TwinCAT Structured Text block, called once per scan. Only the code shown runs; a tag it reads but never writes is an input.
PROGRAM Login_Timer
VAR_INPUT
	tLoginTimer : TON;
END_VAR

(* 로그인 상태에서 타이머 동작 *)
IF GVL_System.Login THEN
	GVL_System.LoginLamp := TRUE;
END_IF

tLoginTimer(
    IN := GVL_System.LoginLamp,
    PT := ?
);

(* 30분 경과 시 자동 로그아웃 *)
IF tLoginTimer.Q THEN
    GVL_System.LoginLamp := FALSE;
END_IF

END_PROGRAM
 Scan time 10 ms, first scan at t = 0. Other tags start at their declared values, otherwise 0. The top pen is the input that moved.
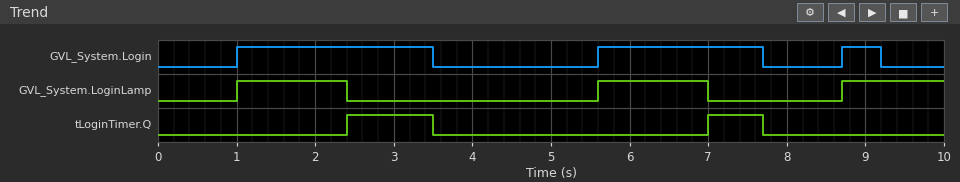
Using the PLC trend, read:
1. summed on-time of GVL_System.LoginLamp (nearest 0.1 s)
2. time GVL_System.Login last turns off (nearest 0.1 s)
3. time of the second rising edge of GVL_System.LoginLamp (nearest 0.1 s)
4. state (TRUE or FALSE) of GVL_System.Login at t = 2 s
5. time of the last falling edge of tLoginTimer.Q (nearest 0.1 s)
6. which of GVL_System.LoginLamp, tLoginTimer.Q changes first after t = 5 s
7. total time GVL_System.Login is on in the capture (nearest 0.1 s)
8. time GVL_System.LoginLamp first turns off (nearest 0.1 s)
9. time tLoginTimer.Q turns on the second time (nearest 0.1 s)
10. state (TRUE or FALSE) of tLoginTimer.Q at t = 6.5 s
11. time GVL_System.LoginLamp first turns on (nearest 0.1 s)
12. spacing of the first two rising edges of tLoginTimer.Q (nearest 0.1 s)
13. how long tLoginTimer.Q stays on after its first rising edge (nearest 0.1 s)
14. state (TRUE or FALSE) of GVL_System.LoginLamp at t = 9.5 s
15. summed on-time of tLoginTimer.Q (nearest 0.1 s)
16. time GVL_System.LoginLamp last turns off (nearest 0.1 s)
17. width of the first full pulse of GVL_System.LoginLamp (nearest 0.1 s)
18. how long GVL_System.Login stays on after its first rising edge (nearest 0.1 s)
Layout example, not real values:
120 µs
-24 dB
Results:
4.1 s
9.2 s
5.6 s
TRUE
7.7 s
GVL_System.LoginLamp
5.1 s
2.4 s
7.0 s
FALSE
1.0 s
4.6 s
1.1 s
TRUE
1.8 s
7.0 s
1.4 s
2.5 s
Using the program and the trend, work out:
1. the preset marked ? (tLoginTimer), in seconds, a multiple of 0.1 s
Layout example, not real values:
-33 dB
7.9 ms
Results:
1.4 s
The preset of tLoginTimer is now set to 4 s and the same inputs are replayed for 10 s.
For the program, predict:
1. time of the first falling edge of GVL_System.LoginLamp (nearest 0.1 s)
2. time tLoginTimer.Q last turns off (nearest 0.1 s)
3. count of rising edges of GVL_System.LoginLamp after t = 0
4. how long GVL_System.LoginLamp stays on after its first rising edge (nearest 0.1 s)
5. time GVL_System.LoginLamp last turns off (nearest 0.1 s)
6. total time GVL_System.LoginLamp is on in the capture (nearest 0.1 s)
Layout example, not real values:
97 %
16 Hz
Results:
5.0 s
9.6 s
2
4.0 s
9.6 s
8.0 s
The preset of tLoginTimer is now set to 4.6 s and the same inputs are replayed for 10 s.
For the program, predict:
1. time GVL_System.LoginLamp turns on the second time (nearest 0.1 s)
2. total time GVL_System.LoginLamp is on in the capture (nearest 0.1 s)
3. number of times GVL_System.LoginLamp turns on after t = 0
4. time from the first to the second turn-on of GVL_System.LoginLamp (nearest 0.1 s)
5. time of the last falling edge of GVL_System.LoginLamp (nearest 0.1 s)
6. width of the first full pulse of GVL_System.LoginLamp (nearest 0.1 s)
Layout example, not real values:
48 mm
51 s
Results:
8.7 s
5.9 s
2
7.7 s
5.6 s
4.6 s
